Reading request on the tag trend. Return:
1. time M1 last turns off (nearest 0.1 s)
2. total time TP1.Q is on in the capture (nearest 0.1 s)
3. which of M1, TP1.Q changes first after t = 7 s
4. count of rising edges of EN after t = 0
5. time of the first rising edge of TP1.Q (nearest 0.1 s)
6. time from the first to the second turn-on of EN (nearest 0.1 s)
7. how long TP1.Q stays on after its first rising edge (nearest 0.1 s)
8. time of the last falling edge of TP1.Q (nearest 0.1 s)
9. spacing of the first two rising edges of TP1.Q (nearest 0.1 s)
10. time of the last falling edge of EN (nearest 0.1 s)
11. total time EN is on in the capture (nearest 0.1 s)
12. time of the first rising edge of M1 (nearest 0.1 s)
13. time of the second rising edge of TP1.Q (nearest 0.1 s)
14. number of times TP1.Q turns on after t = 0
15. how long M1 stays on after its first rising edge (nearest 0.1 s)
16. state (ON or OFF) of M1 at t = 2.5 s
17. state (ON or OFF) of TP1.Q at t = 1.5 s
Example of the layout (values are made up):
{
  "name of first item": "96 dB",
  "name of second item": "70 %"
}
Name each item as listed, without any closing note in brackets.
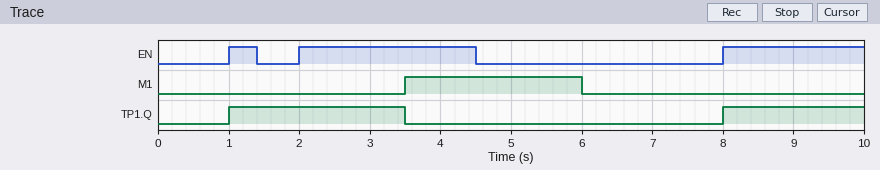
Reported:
{
  "time M1 last turns off": "6.0 s",
  "total time TP1.Q is on in the capture": "4.5 s",
  "which of M1, TP1.Q changes first after t = 7 s": "TP1.Q",
  "count of rising edges of EN after t = 0": "3",
  "time of the first rising edge of TP1.Q": "1.0 s",
  "time from the first to the second turn-on of EN": "1.0 s",
  "how long TP1.Q stays on after its first rising edge": "2.5 s",
  "time of the last falling edge of TP1.Q": "3.5 s",
  "spacing of the first two rising edges of TP1.Q": "7.0 s",
  "time of the last falling edge of EN": "4.5 s",
  "total time EN is on in the capture": "4.9 s",
  "time of the first rising edge of M1": "3.5 s",
  "time of the second rising edge of TP1.Q": "8.0 s",
  "number of times TP1.Q turns on after t = 0": "2",
  "how long M1 stays on after its first rising edge": "2.5 s",
  "state (ON or OFF) of M1 at t = 2.5 s": "OFF",
  "state (ON or OFF) of TP1.Q at t = 1.5 s": "ON"
}
